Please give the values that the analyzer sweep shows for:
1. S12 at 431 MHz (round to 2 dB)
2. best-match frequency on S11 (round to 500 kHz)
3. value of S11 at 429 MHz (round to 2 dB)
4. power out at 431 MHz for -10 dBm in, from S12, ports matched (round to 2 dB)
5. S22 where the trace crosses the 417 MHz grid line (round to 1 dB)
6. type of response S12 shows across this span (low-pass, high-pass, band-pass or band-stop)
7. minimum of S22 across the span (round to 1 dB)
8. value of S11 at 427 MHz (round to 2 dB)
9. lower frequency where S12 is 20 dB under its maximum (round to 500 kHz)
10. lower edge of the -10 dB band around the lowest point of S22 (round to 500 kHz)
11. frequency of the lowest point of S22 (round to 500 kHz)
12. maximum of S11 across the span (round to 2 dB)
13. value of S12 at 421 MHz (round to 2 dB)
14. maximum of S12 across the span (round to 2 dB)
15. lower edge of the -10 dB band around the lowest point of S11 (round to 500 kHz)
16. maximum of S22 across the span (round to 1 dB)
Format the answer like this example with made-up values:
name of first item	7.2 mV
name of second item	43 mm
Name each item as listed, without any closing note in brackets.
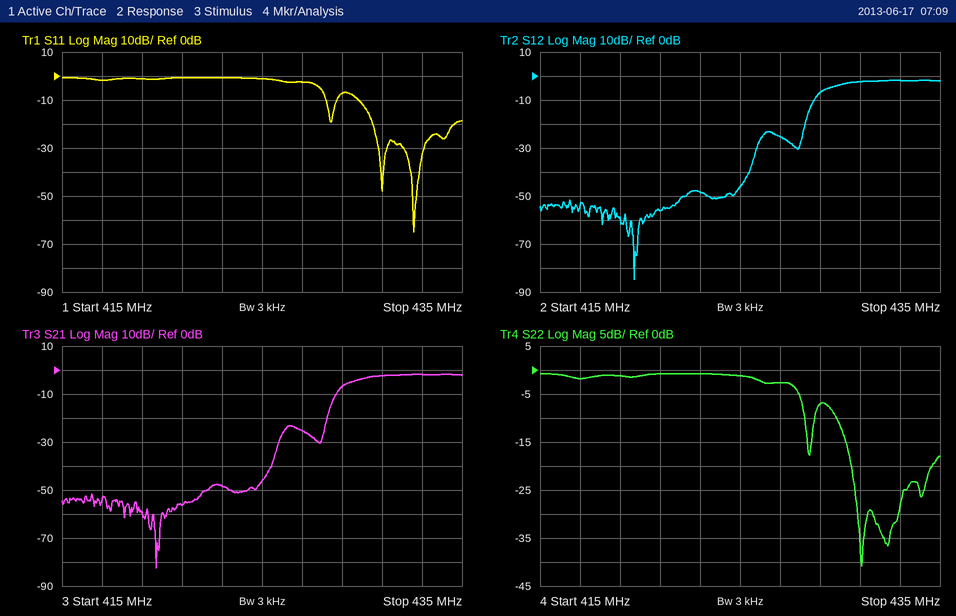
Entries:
S12 at 431 MHz	-2 dB
best-match frequency on S11	432.5 MHz
value of S11 at 429 MHz	-8 dB
power out at 431 MHz for -10 dBm in, from S12, ports matched	-12 dBm
S22 where the trace crosses the 417 MHz grid line	-2 dB
type of response S12 shows across this span	high-pass
minimum of S22 across the span	-41 dB
value of S11 at 427 MHz	-2 dB
lower frequency where S12 is 20 dB under its maximum	428.0 MHz
lower edge of the -10 dB band around the lowest point of S22	430.0 MHz
frequency of the lowest point of S22	431.0 MHz
maximum of S11 across the span	0 dB
value of S12 at 421 MHz	-56 dB
maximum of S12 across the span	-2 dB
lower edge of the -10 dB band around the lowest point of S11	430.0 MHz
maximum of S22 across the span	-1 dB
